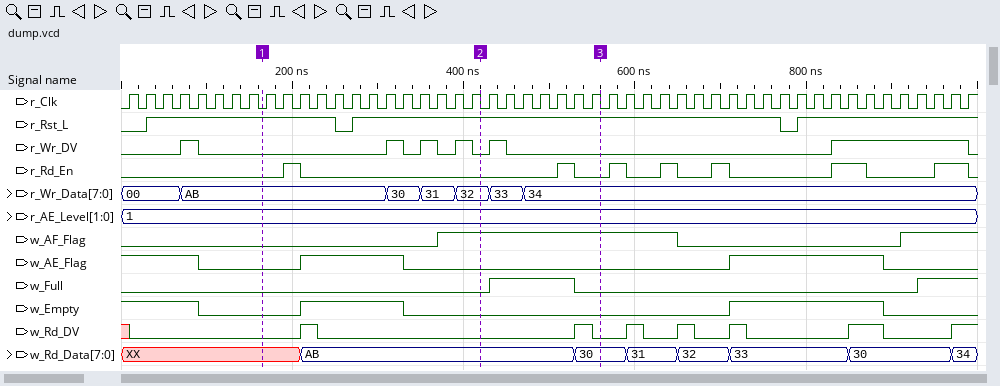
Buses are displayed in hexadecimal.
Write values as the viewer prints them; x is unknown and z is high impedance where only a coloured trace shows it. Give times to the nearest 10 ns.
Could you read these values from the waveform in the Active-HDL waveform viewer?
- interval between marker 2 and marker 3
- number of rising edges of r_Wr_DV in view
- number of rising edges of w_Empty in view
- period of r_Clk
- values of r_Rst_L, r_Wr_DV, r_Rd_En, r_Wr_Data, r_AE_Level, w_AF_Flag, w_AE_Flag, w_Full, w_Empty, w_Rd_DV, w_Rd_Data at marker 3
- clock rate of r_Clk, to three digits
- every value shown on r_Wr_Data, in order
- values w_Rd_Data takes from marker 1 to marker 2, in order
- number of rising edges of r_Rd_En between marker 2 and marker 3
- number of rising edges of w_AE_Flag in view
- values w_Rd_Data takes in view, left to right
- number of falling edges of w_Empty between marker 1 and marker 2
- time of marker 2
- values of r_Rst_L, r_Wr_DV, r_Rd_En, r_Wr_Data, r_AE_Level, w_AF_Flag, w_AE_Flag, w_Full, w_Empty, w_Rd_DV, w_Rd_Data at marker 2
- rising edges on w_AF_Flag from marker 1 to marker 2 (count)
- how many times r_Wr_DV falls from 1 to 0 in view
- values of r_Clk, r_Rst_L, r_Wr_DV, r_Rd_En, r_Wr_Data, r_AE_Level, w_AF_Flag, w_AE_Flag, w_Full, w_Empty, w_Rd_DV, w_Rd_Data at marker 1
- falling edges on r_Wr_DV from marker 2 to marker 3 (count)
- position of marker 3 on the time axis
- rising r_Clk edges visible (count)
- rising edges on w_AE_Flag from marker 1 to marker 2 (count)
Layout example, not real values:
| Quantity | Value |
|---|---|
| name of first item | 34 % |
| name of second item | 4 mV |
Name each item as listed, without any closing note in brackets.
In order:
| Quantity | Value |
|---|---|
| interval between marker 2 and marker 3 | 140 ns |
| number of rising edges of r_Wr_DV in view | 6 |
| number of rising edges of w_Empty in view | 2 |
| period of r_Clk | 20 ns |
| values of r_Rst_L, r_Wr_DV, r_Rd_En, r_Wr_Data, r_AE_Level, w_AF_Flag, w_AE_Flag, w_Full, w_Empty, w_Rd_DV, w_Rd_Data at marker 3 | r_Rst_L=1, r_Wr_DV=0, r_Rd_En=0, r_Wr_Data=34, r_AE_Level=1, w_AF_Flag=1, w_AE_Flag=0, w_Full=0, w_Empty=0, w_Rd_DV=0, w_Rd_Data=30 |
| clock rate of r_Clk, to three digits | 50.0 MHz |
| every value shown on r_Wr_Data, in order | 00, AB, 30, 31, 32, 33, 34 |
| values w_Rd_Data takes from marker 1 to marker 2, in order | XX, AB |
| number of rising edges of r_Rd_En between marker 2 and marker 3 | 1 |
| number of rising edges of w_AE_Flag in view | 2 |
| values w_Rd_Data takes in view, left to right | XX, AB, 30, 31, 32, 33, 30, 34 |
| number of falling edges of w_Empty between marker 1 and marker 2 | 1 |
| time of marker 2 | 420 ns |
| values of r_Rst_L, r_Wr_DV, r_Rd_En, r_Wr_Data, r_AE_Level, w_AF_Flag, w_AE_Flag, w_Full, w_Empty, w_Rd_DV, w_Rd_Data at marker 2 | r_Rst_L=1, r_Wr_DV=0, r_Rd_En=0, r_Wr_Data=32, r_AE_Level=1, w_AF_Flag=1, w_AE_Flag=0, w_Full=0, w_Empty=0, w_Rd_DV=0, w_Rd_Data=AB |
| rising edges on w_AF_Flag from marker 1 to marker 2 | 1 |
| how many times r_Wr_DV falls from 1 to 0 in view | 6 |
| values of r_Clk, r_Rst_L, r_Wr_DV, r_Rd_En, r_Wr_Data, r_AE_Level, w_AF_Flag, w_AE_Flag, w_Full, w_Empty, w_Rd_DV, w_Rd_Data at marker 1 | r_Clk=0, r_Rst_L=1, r_Wr_DV=0, r_Rd_En=0, r_Wr_Data=AB, r_AE_Level=1, w_AF_Flag=0, w_AE_Flag=0, w_Full=0, w_Empty=0, w_Rd_DV=0, w_Rd_Data=XX |
| falling edges on r_Wr_DV from marker 2 to marker 3 | 1 |
| position of marker 3 on the time axis | 560 ns |
| rising r_Clk edges visible | 50 |
| rising edges on w_AE_Flag from marker 1 to marker 2 | 1 |
